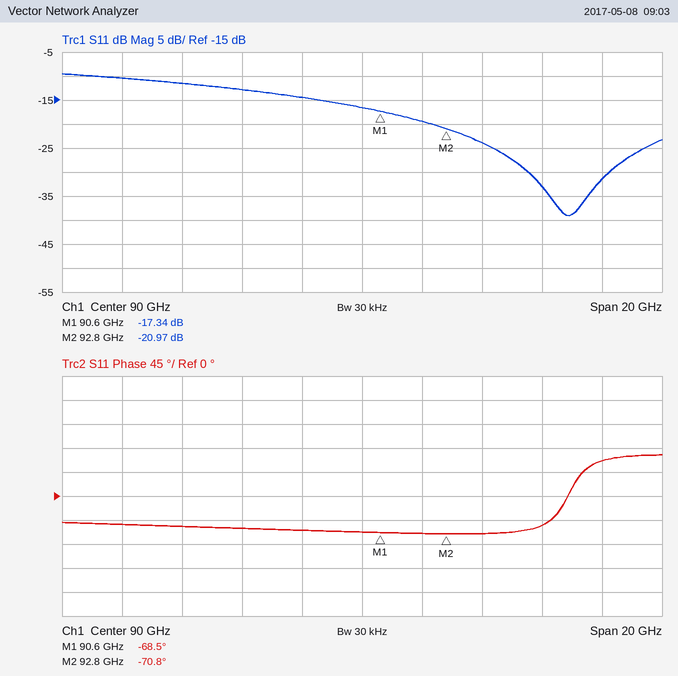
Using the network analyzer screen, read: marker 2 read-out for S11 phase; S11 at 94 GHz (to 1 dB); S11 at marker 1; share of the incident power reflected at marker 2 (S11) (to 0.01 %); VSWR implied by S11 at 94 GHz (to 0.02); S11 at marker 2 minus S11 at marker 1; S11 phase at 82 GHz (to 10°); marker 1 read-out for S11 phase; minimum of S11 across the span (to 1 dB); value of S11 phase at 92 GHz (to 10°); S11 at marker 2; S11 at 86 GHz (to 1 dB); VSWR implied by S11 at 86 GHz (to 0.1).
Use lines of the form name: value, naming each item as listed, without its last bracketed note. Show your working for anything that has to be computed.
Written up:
marker 2 read-out for S11 phase: -70.8°
S11 at 94 GHz: -24 dB
S11 at marker 1: -17.34 dB
share of the incident power reflected at marker 2 (S11): 10^(-20.97/10) ≈ 0.80 %
VSWR implied by S11 at 94 GHz: |Γ| = 10^(-24/20) = 0.0631; VSWR = (1 + 0.0631)/(1 − 0.0631) ≈ 1.13, so 1.14 to the nearest 0.02
S11 at marker 2 minus S11 at marker 1: -20.97 − (-17.34) = -3.63 dB
S11 phase at 82 GHz: -50°
marker 1 read-out for S11 phase: -68.5°
minimum of S11 across the span: -39 dB
value of S11 phase at 92 GHz: -70°
S11 at marker 2: -20.97 dB
S11 at 86 GHz: -13 dB
VSWR implied by S11 at 86 GHz: |Γ| = 10^(-13/20) = 0.2239; VSWR = (1 + 0.2239)/(1 − 0.2239) ≈ 1.6
